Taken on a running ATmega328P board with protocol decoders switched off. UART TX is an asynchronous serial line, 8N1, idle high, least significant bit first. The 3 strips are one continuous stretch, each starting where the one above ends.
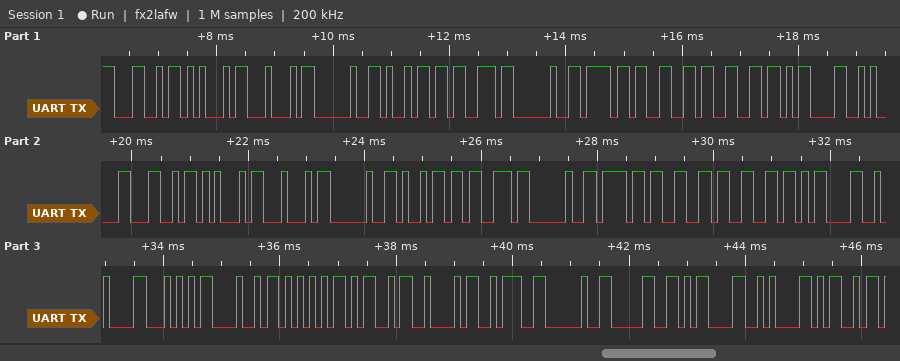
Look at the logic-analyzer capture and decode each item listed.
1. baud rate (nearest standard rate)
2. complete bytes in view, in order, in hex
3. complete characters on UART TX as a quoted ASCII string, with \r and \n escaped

9600 baud
4C 45 44 20 69 73 20 6F 66 66 0D 0A 4C 45 44 20 69 73 20 6F 66 66 0D 0A 54 48 55 4D 42 3A 20 30 0D 0A 4D
"LED is off\r\nLED is off\r\nTHUMB: 0\r\nM"
